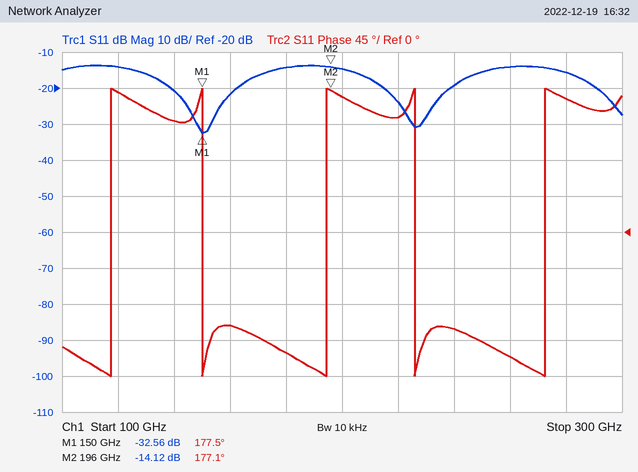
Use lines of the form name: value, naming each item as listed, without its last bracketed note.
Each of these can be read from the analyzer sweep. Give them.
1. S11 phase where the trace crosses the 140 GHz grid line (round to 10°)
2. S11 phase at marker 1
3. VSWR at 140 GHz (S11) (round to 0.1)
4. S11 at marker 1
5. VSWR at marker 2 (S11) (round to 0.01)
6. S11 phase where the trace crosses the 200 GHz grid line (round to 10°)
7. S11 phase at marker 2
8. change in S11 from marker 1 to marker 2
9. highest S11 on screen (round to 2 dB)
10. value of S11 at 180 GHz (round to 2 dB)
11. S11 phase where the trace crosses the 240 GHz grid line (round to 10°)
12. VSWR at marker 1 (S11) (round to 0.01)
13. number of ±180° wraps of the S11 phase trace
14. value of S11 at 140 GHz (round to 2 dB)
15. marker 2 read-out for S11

S11 phase where the trace crosses the 140 GHz grid line: 140°
S11 phase at marker 1: 177.5°
VSWR at 140 GHz (S11): 1.2
S11 at marker 1: -32.56 dB
VSWR at marker 2 (S11): 1.49
S11 phase where the trace crosses the 200 GHz grid line: 170°
S11 phase at marker 2: 177.1°
change in S11 from marker 1 to marker 2: 18.44 dB
highest S11 on screen: -14 dB
value of S11 at 180 GHz: -14 dB
S11 phase where the trace crosses the 240 GHz grid line: -120°
VSWR at marker 1 (S11): 1.05
number of ±180° wraps of the S11 phase trace: 5
value of S11 at 140 GHz: -20 dB
marker 2 read-out for S11: -14.12 dB
